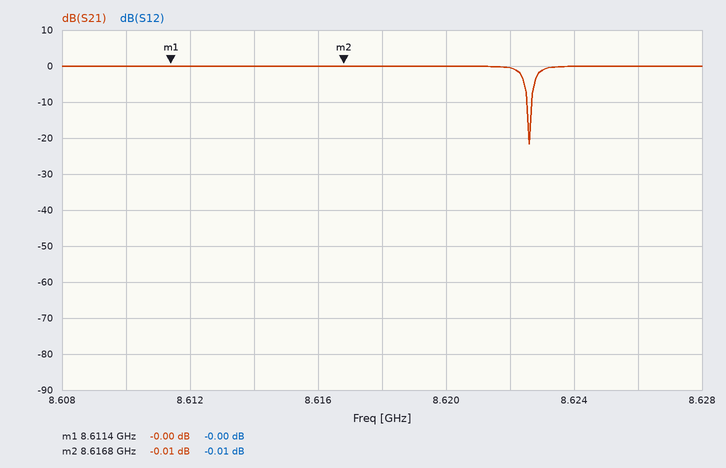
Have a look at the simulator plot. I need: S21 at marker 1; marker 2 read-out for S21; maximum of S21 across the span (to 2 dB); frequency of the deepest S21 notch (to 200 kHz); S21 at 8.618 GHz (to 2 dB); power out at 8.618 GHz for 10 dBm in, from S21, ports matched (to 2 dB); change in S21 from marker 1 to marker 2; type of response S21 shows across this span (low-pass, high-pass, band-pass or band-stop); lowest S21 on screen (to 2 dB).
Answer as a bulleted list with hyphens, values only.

- -0.00 dB
- -0.01 dB
- 0 dB
- 8.6226 GHz
- 0 dB
- 10 dBm
- -0.01 dB
- band-stop
- -22 dB
